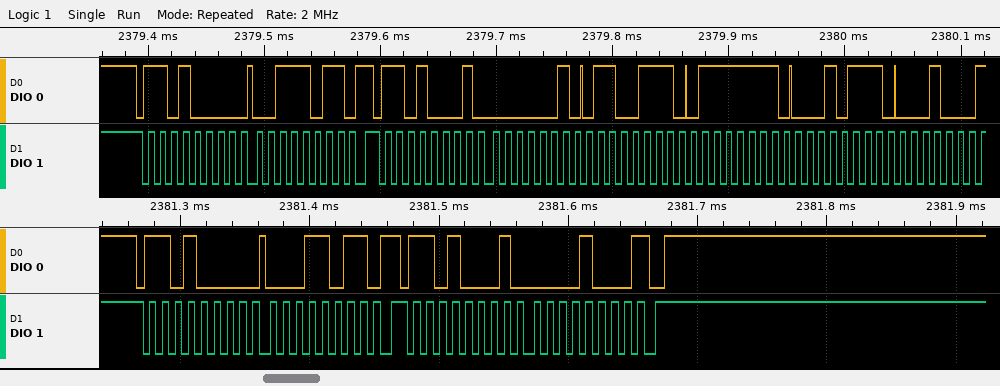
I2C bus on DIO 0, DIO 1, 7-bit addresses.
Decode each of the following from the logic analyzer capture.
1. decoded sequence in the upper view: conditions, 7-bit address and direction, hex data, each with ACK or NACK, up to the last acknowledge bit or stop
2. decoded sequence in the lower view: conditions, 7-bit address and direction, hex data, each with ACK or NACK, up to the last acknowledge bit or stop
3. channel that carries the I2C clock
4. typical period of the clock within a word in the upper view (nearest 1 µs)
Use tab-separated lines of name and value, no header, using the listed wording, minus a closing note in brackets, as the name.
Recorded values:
decoded sequence in the upper view: conditions, 7-bit address and direction, hex data, each with ACK or NACK, up to the last acknowledge bit or stop	start, address 68 write ACK, 3B ACK, repeated start, address 68 read ACK, 02 ACK, CE ACK, FE ACK, 2E ACK
decoded sequence in the lower view: conditions, 7-bit address and direction, hex data, each with ACK or NACK, up to the last acknowledge bit or stop	start, address 68 write ACK, 1B ACK, repeated start, address 68 read ACK, 08 NACK, stop
channel that carries the I2C clock	DIO 1
typical period of the clock within a word in the upper view	10 µs
